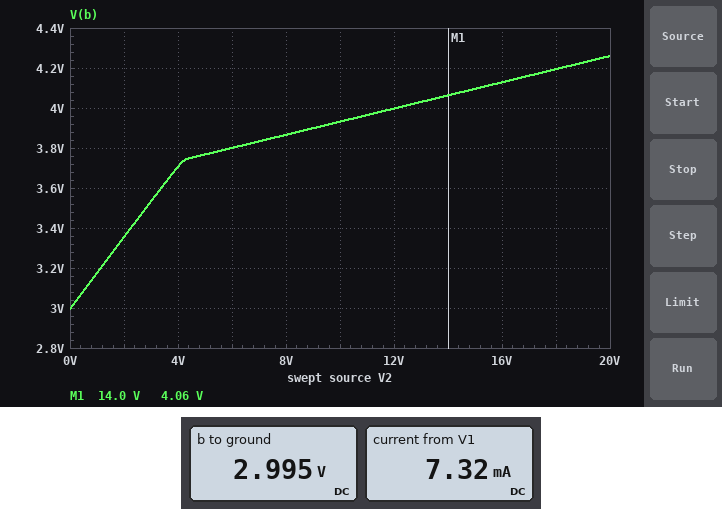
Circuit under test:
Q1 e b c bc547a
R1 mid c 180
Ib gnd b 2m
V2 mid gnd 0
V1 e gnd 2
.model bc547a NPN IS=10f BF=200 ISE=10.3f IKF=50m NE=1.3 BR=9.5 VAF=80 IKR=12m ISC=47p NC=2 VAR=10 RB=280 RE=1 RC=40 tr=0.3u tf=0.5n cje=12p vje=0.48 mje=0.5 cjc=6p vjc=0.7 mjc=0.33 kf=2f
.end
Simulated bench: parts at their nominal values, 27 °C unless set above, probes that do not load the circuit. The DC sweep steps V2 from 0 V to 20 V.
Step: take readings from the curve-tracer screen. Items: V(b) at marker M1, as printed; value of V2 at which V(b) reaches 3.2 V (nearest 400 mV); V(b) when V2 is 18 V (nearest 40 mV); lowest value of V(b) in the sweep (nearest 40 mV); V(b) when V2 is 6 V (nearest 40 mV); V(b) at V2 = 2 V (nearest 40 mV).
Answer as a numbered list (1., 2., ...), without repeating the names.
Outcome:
1. 4.06 V
2. 1.2 V
3. 4.20 V
4. 3.00 V
5. 3.80 V
6. 3.36 V
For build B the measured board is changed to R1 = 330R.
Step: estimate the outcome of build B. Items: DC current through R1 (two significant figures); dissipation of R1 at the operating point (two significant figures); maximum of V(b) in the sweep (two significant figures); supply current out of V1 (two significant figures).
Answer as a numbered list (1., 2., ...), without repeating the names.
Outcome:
1. 5.6 mA
2. 10 mW
3. 4.2 V
4. 3.6 mA
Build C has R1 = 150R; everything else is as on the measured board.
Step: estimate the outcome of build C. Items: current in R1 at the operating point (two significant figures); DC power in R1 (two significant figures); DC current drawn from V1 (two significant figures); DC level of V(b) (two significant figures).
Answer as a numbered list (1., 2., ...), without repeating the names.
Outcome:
1. 11 mA
2. 17 mW
3. 8.8 mA
4. 2.9 V
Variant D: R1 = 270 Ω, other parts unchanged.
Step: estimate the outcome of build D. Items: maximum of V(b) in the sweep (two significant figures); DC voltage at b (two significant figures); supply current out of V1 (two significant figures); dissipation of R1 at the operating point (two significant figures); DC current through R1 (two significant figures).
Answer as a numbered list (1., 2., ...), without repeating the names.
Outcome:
1. 4.2 V
2. 3.1 V
3. 4.6 mA
4. 12 mW
5. 6.6 mA
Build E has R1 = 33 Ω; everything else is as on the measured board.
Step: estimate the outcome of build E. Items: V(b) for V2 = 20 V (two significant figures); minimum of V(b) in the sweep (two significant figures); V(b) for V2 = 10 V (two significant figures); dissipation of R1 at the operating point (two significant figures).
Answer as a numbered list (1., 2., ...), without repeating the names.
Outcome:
1. 4.4 V
2. 2.3 V
3. 4.0 V
4. 25 mW
